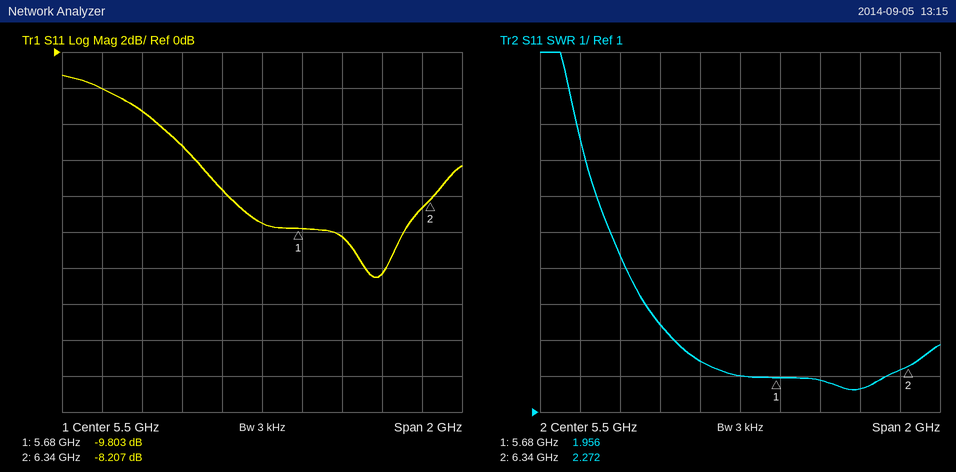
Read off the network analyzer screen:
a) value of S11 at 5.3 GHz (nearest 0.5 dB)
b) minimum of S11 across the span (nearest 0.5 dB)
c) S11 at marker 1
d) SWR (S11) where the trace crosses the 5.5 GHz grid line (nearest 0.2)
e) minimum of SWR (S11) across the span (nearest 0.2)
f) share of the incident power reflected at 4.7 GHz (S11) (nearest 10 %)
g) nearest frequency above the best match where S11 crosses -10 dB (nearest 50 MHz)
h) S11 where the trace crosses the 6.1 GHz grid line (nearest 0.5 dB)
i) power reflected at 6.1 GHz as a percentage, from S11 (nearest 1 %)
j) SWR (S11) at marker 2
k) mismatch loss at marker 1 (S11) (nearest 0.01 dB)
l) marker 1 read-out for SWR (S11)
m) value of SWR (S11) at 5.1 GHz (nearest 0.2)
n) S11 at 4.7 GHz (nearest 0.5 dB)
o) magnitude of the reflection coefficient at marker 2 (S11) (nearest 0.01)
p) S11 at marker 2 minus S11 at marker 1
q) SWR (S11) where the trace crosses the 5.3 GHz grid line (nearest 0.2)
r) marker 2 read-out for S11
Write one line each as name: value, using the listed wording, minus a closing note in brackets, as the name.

value of S11 at 5.3 GHz: -7.5 dB
minimum of S11 across the span: -12.5 dB
S11 at marker 1: -9.803 dB
SWR (S11) where the trace crosses the 5.5 GHz grid line: 2.0
minimum of SWR (S11) across the span: 1.6
share of the incident power reflected at 4.7 GHz (S11): 60 %
nearest frequency above the best match where S11 crosses -10 dB: 6.20 GHz
S11 where the trace crosses the 6.1 GHz grid line: -12.5 dB
power reflected at 6.1 GHz as a percentage, from S11: 6 %
SWR (S11) at marker 2: 2.272
mismatch loss at marker 1 (S11): 0.48 dB
marker 1 read-out for SWR: 1.956
value of SWR (S11) at 5.1 GHz: 3.4
S11 at 4.7 GHz: -2.0 dB
magnitude of the reflection coefficient at marker 2 (S11): 0.39
S11 at marker 2 minus S11 at marker 1: 1.596 dB
SWR (S11) where the trace crosses the 5.3 GHz grid line: 2.4
marker 2 read-out for S11: -8.207 dB
